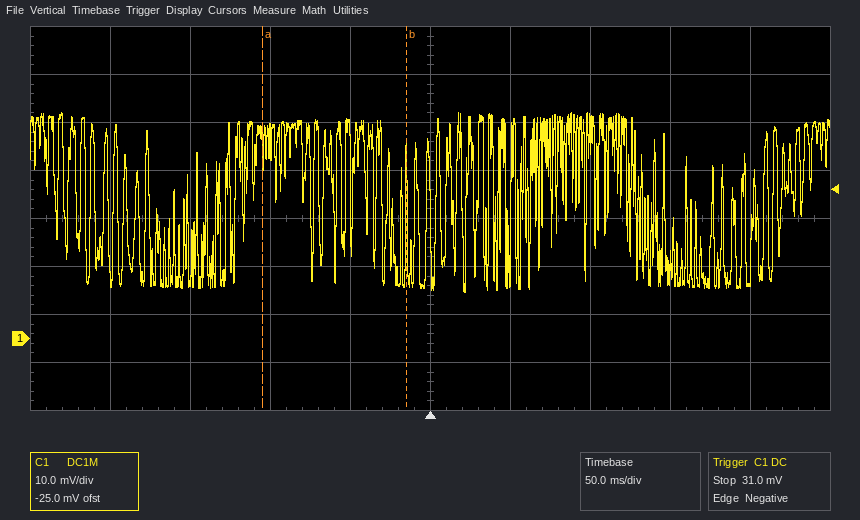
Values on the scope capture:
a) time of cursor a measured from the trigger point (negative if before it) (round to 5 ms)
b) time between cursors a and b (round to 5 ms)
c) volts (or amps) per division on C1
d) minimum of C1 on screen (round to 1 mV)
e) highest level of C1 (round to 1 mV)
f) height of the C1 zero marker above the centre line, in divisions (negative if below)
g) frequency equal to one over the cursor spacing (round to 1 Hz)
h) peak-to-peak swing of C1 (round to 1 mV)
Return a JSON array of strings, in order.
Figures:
["-105 ms", "90 ms", "10 mV", "10 mV", "47 mV", "-2.5 div", "11 Hz", "37 mV"]
